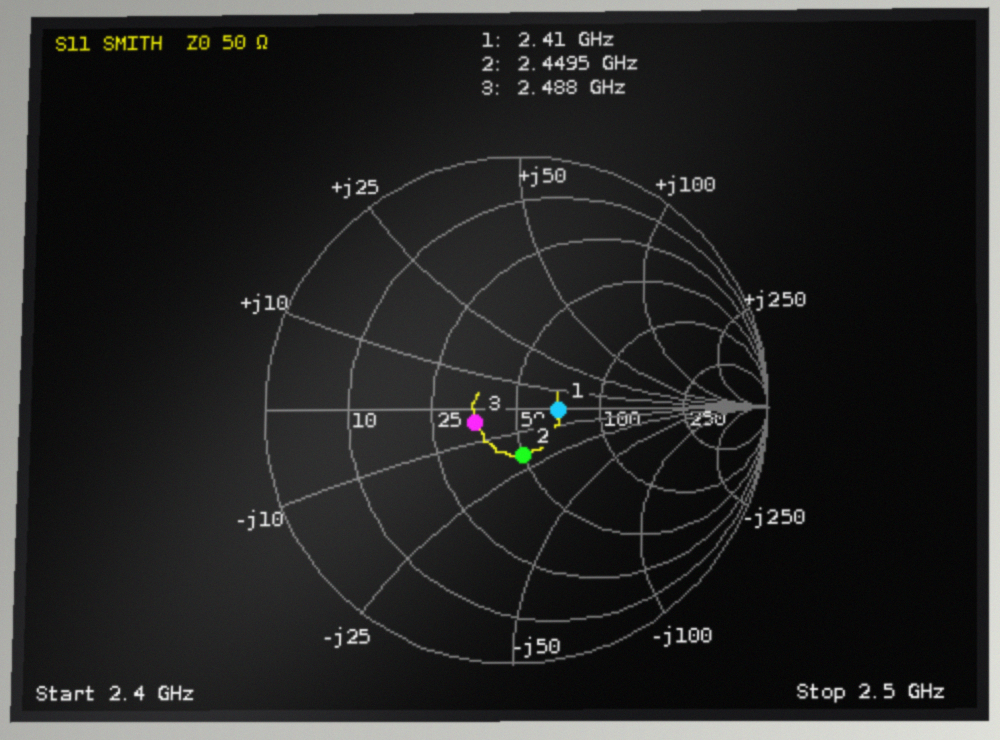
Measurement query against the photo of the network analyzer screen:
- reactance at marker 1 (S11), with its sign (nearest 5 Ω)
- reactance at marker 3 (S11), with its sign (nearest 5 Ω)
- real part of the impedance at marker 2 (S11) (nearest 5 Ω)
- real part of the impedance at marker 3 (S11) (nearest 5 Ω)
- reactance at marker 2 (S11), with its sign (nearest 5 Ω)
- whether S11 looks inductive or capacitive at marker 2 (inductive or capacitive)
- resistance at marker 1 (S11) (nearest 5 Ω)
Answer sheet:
0 Ω
-5 Ω
50 Ω
35 Ω
-20 Ω
capacitive
70 Ω
